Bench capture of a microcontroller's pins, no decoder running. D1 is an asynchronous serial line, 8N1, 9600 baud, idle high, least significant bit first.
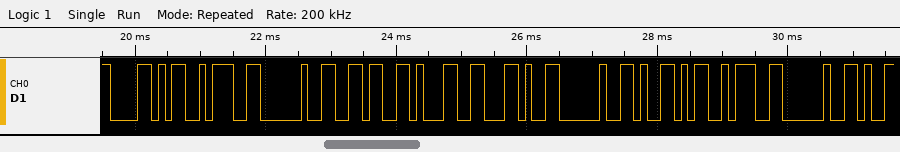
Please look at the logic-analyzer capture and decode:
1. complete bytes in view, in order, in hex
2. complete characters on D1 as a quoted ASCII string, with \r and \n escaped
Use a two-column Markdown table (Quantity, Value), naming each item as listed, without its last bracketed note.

| Quantity | Value |
|---|---|
| complete bytes in view, in order, in hex | 0x58 0x3A 0x20 0x36 0x31 0x2C 0x20 0x59 0x3A 0x20 |
| complete characters on D1 as a quoted ASCII string, with \r and \n escaped | "X: 61, Y: " |
